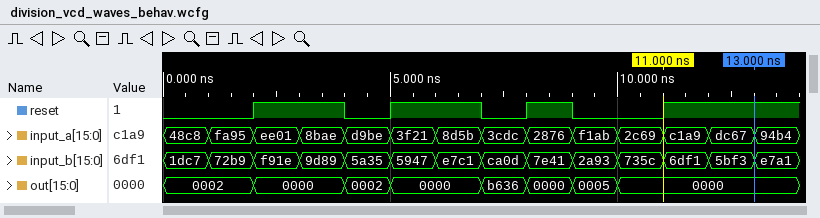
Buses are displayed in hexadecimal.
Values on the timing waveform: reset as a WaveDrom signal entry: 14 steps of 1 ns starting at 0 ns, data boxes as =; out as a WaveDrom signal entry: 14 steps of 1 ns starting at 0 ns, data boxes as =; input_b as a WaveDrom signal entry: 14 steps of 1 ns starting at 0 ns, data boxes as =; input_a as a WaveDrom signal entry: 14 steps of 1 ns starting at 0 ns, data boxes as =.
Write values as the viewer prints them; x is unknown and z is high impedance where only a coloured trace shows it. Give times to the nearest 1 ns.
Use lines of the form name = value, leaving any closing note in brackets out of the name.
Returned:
reset as a WaveDrom signal entry: 14 steps of 1 ns starting at 0 ns, data boxes as = = {name: 'reset', wave: '0.1.01.010.1..'}
out as a WaveDrom signal entry: 14 steps of 1 ns starting at 0 ns, data boxes as = = {name: 'out', wave: '=.=.==.====...', data: '0002 0000 0002 0000 b636 0000 0005 0000'}
input_b as a WaveDrom signal entry: 14 steps of 1 ns starting at 0 ns, data boxes as = = {name: 'input_b', wave: '==============', data: '1dc7 72b9 f91e 9d89 5a35 5947 e7c1 ca0d 7e41 2a93 735c 6df1 5bf3 e7a1'}
input_a as a WaveDrom signal entry: 14 steps of 1 ns starting at 0 ns, data boxes as = = {name: 'input_a', wave: '==============', data: '48c8 fa95 ee01 8bae d9be 3f21 8d5b 3cdc 2876 f1ab 2c69 c1a9 dc67 94b4'}
